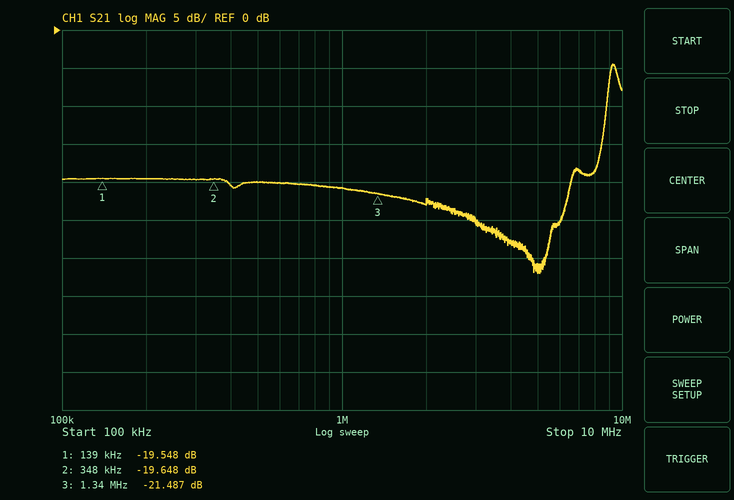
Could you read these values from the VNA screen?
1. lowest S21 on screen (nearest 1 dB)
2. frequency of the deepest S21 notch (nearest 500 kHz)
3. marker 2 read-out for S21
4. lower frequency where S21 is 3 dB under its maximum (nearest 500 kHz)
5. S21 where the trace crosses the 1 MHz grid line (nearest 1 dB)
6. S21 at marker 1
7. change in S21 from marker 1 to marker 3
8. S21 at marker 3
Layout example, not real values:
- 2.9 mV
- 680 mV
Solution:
- -32 dB
- 5.0 MHz
- -19.648 dB
- 9.0 MHz
- -21 dB
- -19.548 dB
- -1.939 dB
- -21.487 dB
